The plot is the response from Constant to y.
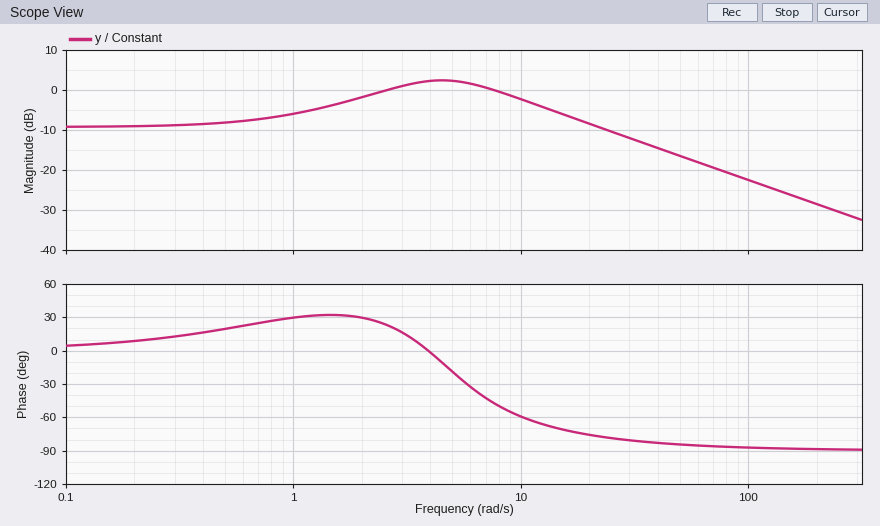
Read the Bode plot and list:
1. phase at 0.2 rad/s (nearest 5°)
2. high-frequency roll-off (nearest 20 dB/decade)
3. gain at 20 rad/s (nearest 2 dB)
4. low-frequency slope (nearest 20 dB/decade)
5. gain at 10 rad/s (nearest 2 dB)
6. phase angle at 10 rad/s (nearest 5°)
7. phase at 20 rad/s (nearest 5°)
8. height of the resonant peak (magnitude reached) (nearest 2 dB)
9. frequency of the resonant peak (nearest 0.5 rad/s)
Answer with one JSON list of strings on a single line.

["10°", "-20 dB/decade", "-8 dB", "0 dB/decade", "-2 dB", "-60°", "-75°", "2 dB", "4.5 rad/s"]
